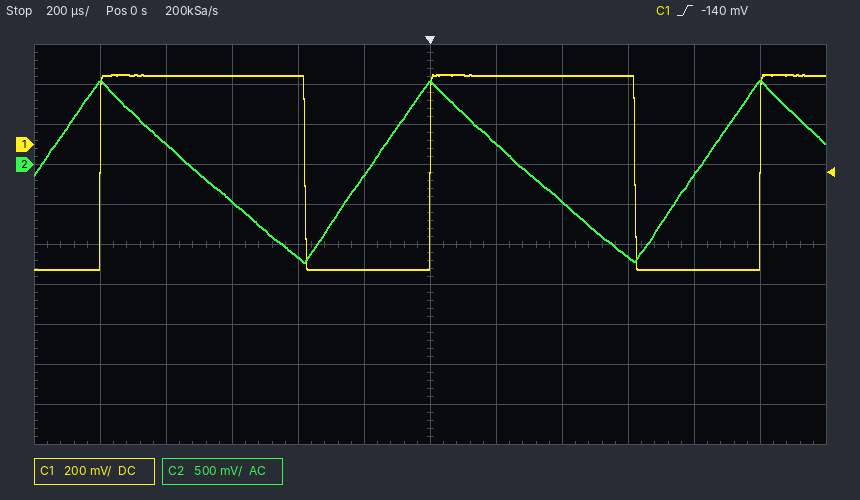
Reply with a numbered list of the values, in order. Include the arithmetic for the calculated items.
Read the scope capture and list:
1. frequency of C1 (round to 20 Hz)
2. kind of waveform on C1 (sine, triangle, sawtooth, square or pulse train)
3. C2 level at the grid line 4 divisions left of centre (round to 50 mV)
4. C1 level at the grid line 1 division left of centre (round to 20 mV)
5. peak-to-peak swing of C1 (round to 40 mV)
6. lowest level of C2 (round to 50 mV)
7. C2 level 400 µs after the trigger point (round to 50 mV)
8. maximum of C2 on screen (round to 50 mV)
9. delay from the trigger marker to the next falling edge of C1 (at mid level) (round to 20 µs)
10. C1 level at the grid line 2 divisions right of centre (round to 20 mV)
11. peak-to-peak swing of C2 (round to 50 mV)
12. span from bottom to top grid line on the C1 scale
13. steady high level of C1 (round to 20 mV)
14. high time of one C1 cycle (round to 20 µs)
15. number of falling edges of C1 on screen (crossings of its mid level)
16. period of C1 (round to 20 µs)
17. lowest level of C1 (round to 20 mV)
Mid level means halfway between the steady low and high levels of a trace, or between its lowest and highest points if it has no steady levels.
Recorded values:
1. 1 / 1.00 ms ≈ 1.00 kHz
2. pulse train
3. 250 mV
4. -620 mV
5. 960 mV
6. -1.20 V
7. -450 mV
8. 1.05 V
9. 620 µs
10. 340 mV
11. 1.05 V − (-1.20 V) = 2.25 V
12. 2 V
13. 340 mV
14. 620 µs
15. 2
16. 1.00 ms
17. -620 mV
